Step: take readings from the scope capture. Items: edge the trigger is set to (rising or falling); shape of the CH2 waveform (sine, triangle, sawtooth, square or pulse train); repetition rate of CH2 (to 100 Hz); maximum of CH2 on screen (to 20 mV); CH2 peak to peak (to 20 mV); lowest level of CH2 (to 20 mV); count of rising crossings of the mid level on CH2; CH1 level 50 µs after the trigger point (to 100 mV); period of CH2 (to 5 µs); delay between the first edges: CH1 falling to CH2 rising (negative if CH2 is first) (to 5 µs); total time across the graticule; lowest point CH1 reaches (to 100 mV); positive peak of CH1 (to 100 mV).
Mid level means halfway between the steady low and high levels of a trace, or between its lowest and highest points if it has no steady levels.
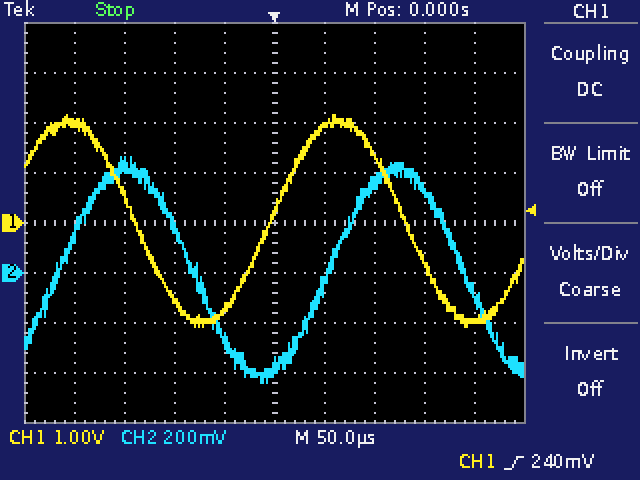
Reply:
rising
sine
3.7 kHz
460 mV
900 mV
-440 mV
2
1.9 V
270 µs
-75 µs
500 µs
-2.1 V
2.2 V
